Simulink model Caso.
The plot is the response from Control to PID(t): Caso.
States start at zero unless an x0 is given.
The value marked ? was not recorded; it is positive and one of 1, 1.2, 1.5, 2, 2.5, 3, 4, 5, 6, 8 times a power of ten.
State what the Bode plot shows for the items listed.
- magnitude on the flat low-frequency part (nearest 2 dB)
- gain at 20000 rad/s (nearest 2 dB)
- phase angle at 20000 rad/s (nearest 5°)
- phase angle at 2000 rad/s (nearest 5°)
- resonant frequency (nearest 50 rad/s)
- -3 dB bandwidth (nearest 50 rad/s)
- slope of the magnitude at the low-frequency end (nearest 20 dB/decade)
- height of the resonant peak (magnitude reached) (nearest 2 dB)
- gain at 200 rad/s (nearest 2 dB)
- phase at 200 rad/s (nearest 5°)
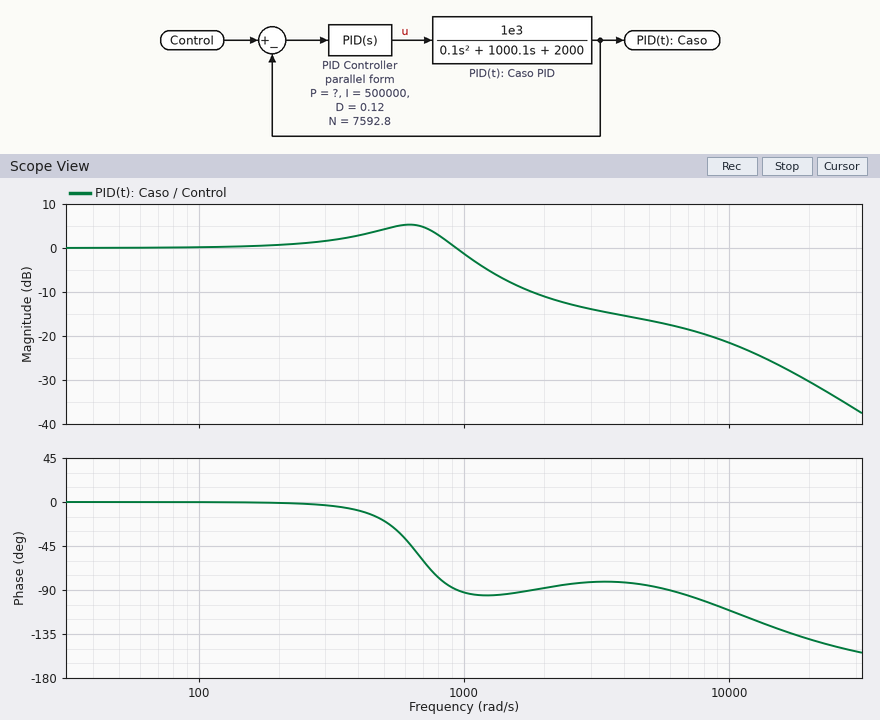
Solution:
0 dB
-30 dB
-140°
-90°
600 rad/s
1100 rad/s
0 dB/decade
6 dB
0 dB
0°
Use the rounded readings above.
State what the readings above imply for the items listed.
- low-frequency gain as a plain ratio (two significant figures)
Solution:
1.0
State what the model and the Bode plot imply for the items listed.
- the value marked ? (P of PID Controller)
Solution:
500
